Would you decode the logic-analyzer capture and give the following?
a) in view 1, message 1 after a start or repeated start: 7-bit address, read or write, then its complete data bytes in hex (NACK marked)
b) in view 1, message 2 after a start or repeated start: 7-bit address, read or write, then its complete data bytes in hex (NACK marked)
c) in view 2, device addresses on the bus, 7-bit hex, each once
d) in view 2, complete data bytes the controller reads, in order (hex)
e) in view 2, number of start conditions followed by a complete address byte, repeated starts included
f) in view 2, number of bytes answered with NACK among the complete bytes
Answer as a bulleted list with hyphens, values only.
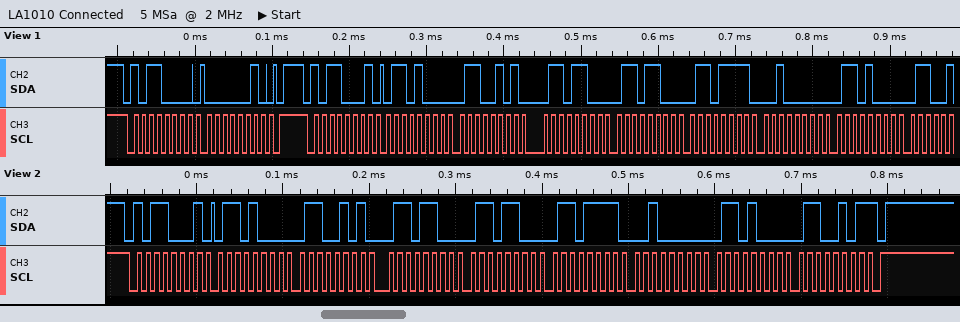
- 0x58 write: 02
- 0x58 read: 68 65 6C 6C 6F 20 68
- 0x58
- 68 65 6C 6C 6F 20 68 65
- 1
- 1
